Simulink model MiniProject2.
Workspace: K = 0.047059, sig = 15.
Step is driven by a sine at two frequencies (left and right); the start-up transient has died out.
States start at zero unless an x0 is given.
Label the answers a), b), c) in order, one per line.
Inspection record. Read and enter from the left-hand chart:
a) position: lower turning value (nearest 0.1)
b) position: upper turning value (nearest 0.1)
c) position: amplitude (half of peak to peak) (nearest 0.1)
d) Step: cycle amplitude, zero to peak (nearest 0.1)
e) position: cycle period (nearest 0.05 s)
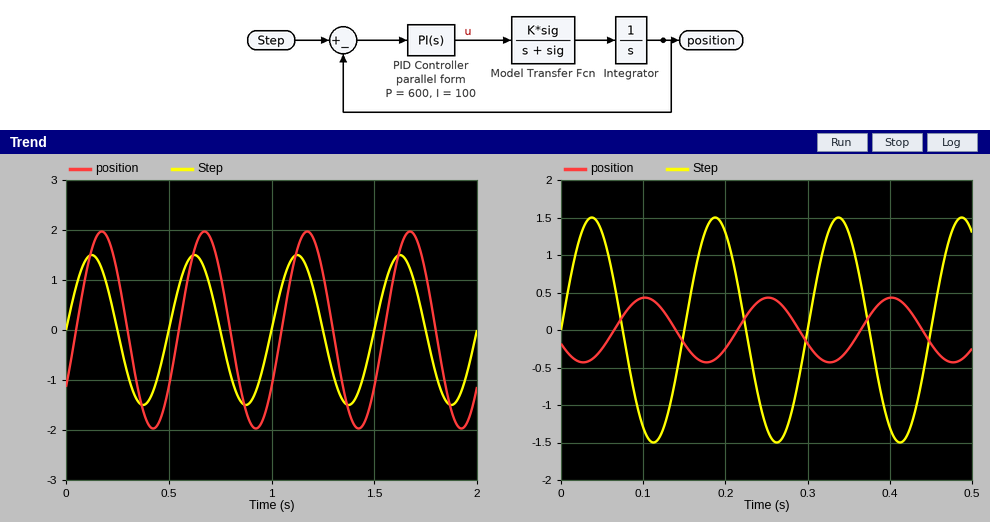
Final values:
a) -2.0
b) 2.0
c) 2.0
d) 1.5
e) 0.50 s
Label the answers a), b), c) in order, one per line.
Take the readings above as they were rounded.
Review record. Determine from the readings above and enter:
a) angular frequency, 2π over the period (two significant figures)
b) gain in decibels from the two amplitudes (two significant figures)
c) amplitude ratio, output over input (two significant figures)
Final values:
a) 13 rad/s
b) 2.5 dB
c) 1.3
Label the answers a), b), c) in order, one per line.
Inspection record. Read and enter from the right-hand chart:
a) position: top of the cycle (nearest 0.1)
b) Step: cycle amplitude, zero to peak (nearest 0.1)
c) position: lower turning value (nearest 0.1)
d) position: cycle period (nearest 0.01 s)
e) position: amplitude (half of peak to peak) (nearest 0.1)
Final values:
a) 0.4
b) 1.5
c) -0.4
d) 0.15 s
e) 0.4
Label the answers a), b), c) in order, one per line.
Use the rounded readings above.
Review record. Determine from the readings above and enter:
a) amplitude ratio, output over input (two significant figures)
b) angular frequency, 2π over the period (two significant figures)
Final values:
a) 0.27
b) 42 rad/s
